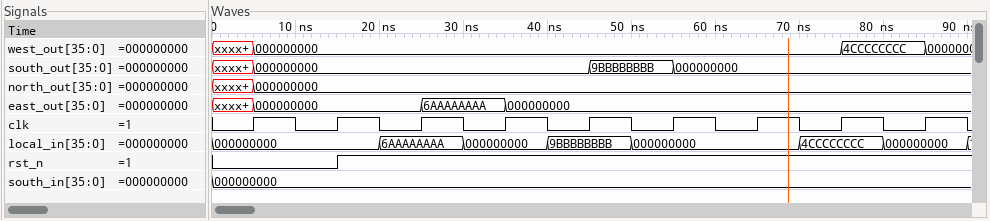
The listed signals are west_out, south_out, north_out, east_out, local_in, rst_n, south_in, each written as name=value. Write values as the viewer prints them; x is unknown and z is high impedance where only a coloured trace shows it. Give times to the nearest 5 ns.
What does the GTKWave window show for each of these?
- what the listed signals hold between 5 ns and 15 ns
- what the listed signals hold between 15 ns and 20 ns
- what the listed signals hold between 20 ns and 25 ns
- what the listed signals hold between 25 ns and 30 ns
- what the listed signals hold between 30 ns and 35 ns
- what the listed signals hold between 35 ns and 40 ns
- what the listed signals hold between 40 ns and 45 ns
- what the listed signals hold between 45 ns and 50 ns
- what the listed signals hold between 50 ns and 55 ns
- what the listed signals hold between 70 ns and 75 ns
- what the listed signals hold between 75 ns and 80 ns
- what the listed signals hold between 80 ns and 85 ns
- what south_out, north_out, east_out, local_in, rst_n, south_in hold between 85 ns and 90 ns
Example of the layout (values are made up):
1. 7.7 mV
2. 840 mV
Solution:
1. west_out=000000000, south_out=000000000, north_out=000000000, east_out=000000000, local_in=000000000, rst_n=0, south_in=000000000
2. west_out=000000000, south_out=000000000, north_out=000000000, east_out=000000000, local_in=000000000, rst_n=1, south_in=000000000
3. west_out=000000000, south_out=000000000, north_out=000000000, east_out=000000000, local_in=6AAAAAAAA, rst_n=1, south_in=000000000
4. west_out=000000000, south_out=000000000, north_out=000000000, east_out=6AAAAAAAA, local_in=6AAAAAAAA, rst_n=1, south_in=000000000
5. west_out=000000000, south_out=000000000, north_out=000000000, east_out=6AAAAAAAA, local_in=000000000, rst_n=1, south_in=000000000
6. west_out=000000000, south_out=000000000, north_out=000000000, east_out=000000000, local_in=000000000, rst_n=1, south_in=000000000
7. west_out=000000000, south_out=000000000, north_out=000000000, east_out=000000000, local_in=9BBBBBBBB, rst_n=1, south_in=000000000
8. west_out=000000000, south_out=9BBBBBBBB, north_out=000000000, east_out=000000000, local_in=9BBBBBBBB, rst_n=1, south_in=000000000
9. west_out=000000000, south_out=9BBBBBBBB, north_out=000000000, east_out=000000000, local_in=000000000, rst_n=1, south_in=000000000
10. west_out=000000000, south_out=000000000, north_out=000000000, east_out=000000000, local_in=4CCCCCCCC, rst_n=1, south_in=000000000
11. west_out=4CCCCCCCC, south_out=000000000, north_out=000000000, east_out=000000000, local_in=4CCCCCCCC, rst_n=1, south_in=000000000
12. west_out=4CCCCCCCC, south_out=000000000, north_out=000000000, east_out=000000000, local_in=000000000, rst_n=1, south_in=000000000
13. south_out=000000000, north_out=000000000, east_out=000000000, local_in=000000000, rst_n=1, south_in=000000000
